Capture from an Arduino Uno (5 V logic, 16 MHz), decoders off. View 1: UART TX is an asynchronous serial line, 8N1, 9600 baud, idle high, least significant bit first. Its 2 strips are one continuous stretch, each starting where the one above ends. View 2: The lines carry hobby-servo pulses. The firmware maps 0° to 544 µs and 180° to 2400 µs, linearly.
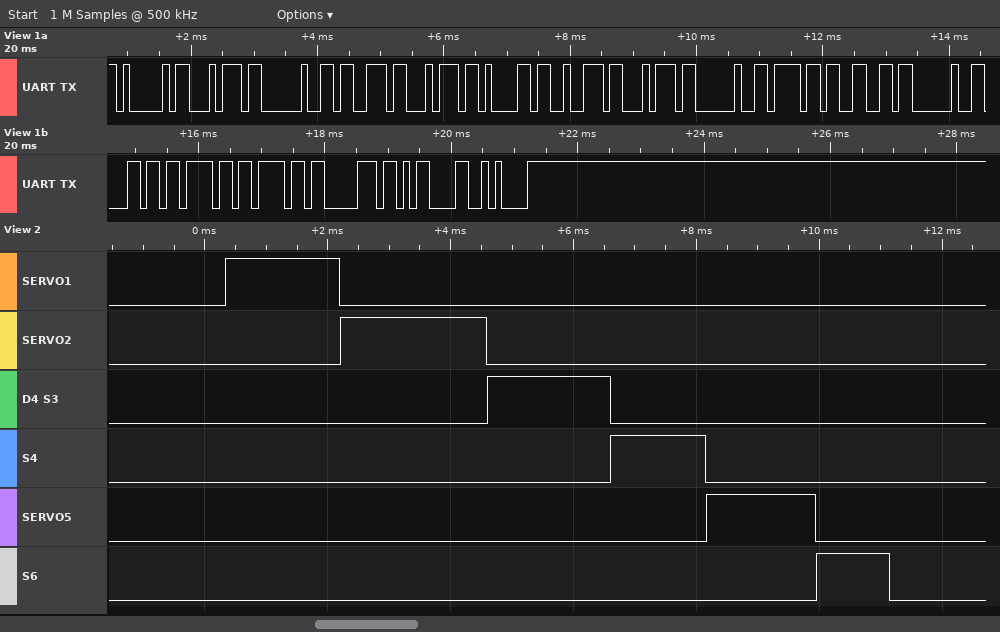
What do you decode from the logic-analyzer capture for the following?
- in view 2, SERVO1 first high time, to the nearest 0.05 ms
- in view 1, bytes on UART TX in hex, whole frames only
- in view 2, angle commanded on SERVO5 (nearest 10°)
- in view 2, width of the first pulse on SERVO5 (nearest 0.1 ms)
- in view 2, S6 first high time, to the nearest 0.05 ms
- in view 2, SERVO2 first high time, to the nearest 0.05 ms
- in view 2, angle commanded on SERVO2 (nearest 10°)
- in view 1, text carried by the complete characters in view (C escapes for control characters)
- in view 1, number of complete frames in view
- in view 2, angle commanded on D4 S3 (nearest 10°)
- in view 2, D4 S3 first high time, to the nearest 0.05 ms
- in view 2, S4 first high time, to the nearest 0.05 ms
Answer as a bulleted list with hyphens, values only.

- 1.85 ms
- 41 74 20 73 74 61 72 74 20 6F 66 20 6C 6F 6F 70 0D 0A
- 120°
- 1.8 ms
- 1.20 ms
- 2.40 ms
- 180°
- "At start of loop\r\n"
- 18
- 140°
- 2.00 ms
- 1.55 ms
